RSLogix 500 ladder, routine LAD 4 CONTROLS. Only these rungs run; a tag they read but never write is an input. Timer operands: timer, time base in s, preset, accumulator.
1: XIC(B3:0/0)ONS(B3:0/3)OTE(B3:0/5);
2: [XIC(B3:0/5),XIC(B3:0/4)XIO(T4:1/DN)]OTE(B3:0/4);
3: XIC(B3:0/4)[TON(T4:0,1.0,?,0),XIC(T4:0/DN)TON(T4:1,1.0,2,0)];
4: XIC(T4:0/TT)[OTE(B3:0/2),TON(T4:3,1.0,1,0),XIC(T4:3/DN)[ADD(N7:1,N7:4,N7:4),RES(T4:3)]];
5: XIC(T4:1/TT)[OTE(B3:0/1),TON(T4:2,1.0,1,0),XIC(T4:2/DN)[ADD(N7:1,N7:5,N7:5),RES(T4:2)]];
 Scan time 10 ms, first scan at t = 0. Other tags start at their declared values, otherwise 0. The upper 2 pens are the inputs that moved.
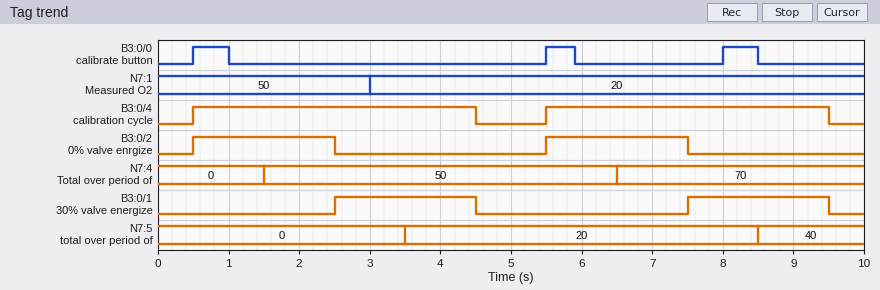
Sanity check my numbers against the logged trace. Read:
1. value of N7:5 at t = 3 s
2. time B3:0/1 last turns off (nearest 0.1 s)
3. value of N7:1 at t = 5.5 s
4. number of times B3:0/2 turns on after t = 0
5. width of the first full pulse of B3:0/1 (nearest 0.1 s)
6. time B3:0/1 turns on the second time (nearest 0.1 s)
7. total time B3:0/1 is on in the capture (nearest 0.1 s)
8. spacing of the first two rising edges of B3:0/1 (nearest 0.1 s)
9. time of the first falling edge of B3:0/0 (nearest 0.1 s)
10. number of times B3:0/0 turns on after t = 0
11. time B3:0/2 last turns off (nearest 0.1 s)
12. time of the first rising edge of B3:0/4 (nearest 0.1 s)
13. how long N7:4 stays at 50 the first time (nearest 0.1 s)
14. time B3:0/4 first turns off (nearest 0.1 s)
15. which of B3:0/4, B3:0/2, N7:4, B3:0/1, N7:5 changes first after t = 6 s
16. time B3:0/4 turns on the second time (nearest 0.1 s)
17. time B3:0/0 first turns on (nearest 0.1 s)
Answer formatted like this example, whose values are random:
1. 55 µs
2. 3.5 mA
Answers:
1. 0
2. 9.5 s
3. 20
4. 2
5. 2.0 s
6. 7.5 s
7. 4.0 s
8. 5.0 s
9. 1.0 s
10. 3
11. 7.5 s
12. 0.5 s
13. 5.0 s
14. 4.5 s
15. N7:4
16. 5.5 s
17. 0.5 s
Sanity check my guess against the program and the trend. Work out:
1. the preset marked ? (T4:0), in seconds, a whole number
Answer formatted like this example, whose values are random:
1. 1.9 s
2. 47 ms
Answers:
1. 2 s
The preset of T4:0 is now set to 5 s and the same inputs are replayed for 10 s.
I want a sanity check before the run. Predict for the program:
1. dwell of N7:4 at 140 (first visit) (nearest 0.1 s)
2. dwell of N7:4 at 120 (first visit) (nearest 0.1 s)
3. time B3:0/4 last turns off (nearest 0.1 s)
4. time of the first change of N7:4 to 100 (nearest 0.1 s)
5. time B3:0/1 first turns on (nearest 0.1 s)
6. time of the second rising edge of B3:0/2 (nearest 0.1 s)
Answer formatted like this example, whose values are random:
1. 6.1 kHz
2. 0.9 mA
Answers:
1. 4.5 s
2. 1.0 s
3. 7.5 s
4. 2.5 s
5. 5.5 s
6. 8.0 s
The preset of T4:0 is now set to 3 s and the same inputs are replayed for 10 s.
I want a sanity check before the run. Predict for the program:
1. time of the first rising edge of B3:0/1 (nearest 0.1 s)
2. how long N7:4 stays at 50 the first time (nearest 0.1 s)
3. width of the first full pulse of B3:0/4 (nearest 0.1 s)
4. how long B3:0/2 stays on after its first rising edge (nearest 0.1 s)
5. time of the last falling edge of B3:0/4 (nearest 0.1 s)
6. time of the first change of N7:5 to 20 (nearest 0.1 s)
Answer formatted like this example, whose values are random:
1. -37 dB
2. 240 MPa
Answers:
1. 3.5 s
2. 1.0 s
3. 5.0 s
4. 3.0 s
5. 5.5 s
6. 4.5 s
